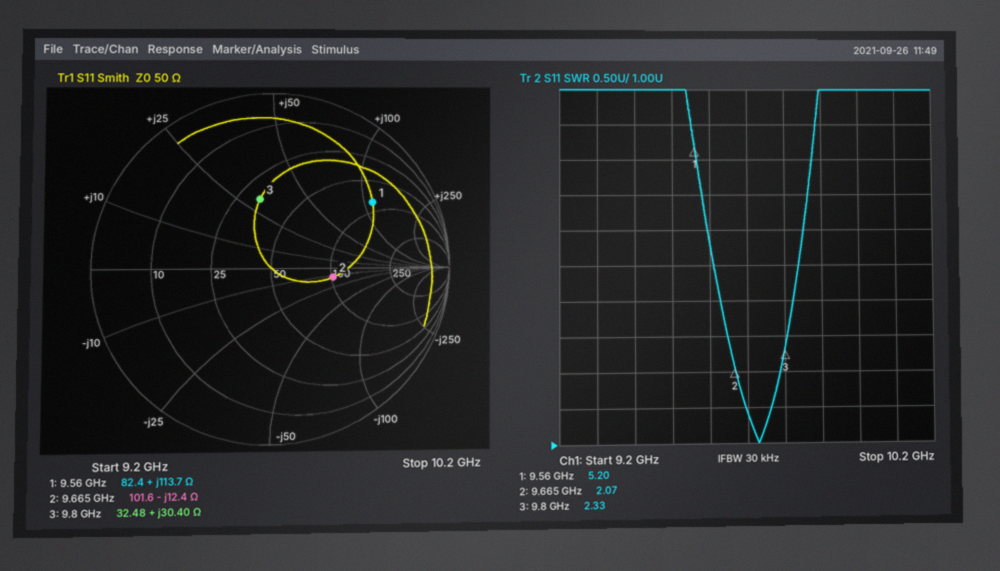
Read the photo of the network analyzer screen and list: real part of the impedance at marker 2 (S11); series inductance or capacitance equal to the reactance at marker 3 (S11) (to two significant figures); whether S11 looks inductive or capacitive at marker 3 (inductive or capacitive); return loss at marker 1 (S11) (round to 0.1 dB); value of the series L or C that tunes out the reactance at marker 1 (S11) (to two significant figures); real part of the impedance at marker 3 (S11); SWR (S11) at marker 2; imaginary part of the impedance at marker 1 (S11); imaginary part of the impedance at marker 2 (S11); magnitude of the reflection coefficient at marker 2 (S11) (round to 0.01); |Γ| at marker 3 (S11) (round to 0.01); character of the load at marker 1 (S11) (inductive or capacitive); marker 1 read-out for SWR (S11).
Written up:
101.6 Ω
490 pH
inductive
3.4 dB
150 fF
32.48 Ω
2.07
+113.7 Ω
-12.4 Ω
0.35
0.40
inductive
5.20
